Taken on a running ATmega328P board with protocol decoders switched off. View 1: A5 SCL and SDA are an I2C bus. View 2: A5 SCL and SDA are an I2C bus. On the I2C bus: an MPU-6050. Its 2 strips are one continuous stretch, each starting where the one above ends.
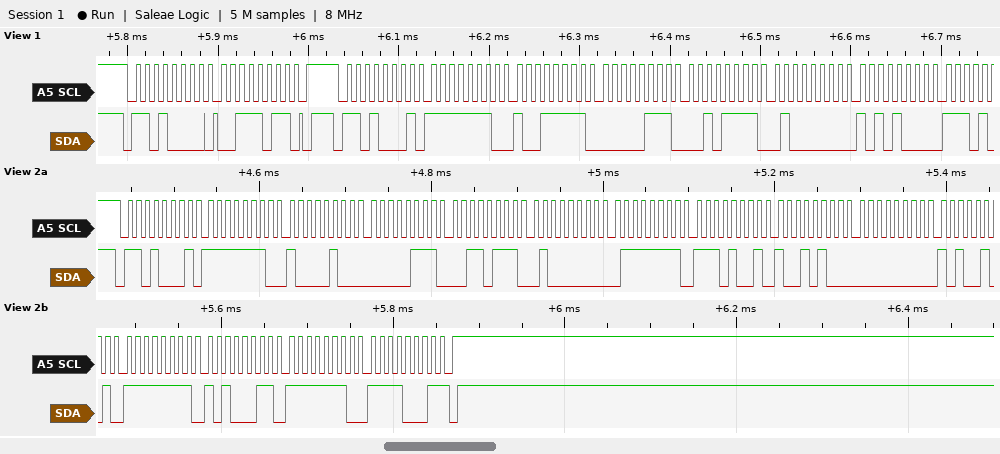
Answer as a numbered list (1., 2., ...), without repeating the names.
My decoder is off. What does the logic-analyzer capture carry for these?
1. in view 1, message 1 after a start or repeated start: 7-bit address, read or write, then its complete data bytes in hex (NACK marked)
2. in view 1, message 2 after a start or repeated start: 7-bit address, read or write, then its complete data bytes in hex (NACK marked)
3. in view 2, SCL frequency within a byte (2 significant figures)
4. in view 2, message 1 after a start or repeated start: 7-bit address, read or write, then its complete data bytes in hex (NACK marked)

1. 0x68 write: 3B
2. 0x68 read: FE 9F 07 2F 40 A8
3. 100 kHz
4. 0x68 read: FE 84 07 37 40 7F E9 94 00 A5 FF A3 FE F1 NACK
